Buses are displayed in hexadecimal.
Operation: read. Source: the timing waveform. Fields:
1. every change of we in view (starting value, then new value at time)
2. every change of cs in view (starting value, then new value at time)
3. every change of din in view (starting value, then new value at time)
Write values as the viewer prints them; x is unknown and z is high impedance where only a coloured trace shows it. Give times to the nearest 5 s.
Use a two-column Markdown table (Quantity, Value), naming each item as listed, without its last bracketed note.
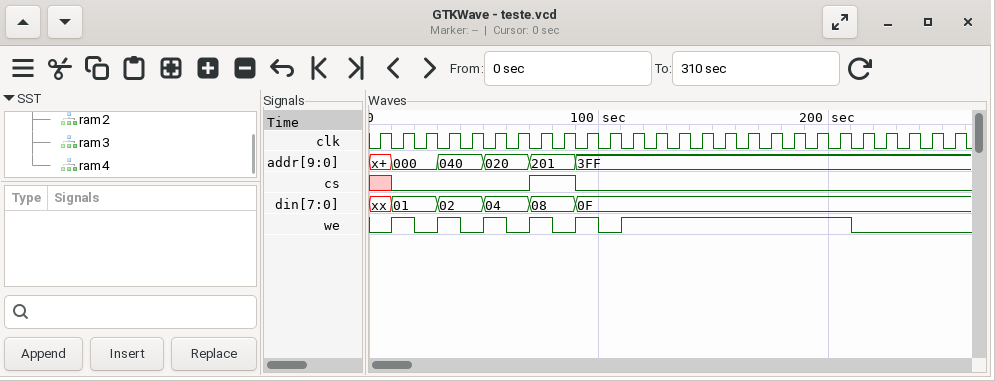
| Quantity | Value |
|---|---|
| every change of we in view | 0, 1 at 10 s, 0 at 20 s, 1 at 30 s, 0 at 40 s, 1 at 50 s, 0 at 60 s, 1 at 70 s, 0 at 80 s, 1 at 90 s, 0 at 100 s, 1 at 110 s, 0 at 210 s |
| every change of cs in view | x, 0 at 10 s, 1 at 70 s, 0 at 90 s |
| every change of din in view | xx, 01 at 10 s, 02 at 30 s, 04 at 50 s, 08 at 70 s, 0F at 90 s |
